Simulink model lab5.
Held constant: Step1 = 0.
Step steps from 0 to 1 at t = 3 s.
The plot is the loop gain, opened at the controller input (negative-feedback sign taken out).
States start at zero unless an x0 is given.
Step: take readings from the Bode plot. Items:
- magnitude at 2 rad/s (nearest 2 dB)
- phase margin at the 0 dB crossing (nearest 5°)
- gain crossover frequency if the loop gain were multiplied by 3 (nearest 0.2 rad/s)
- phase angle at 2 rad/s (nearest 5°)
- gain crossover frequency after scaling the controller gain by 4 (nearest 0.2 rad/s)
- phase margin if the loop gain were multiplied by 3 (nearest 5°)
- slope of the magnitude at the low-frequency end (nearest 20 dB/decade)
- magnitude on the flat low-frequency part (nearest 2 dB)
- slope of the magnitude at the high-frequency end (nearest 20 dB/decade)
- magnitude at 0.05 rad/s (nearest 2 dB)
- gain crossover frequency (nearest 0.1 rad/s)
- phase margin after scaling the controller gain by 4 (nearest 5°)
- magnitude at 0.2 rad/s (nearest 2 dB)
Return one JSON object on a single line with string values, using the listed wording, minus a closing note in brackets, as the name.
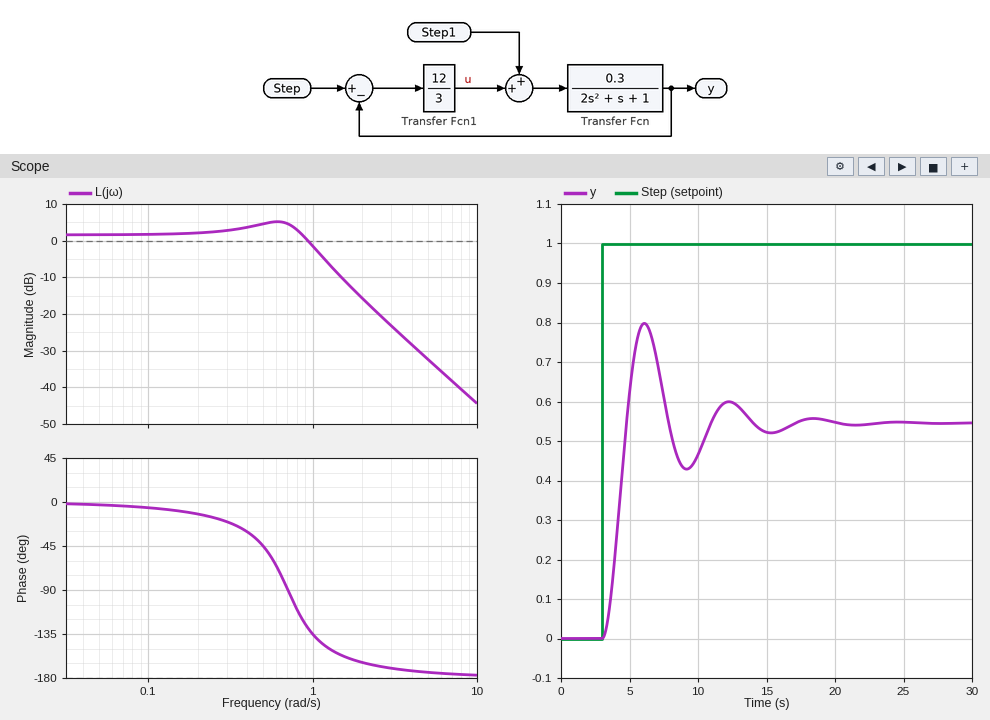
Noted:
{"magnitude at 2 rad/s": "-16 dB", "phase margin at the 0 dB crossing": "50°", "gain crossover frequency if the loop gain were multiplied by 3": "1.4 rad/s", "phase angle at 2 rad/s": "-165°", "gain crossover frequency after scaling the controller gain by 4": "1.6 rad/s", "phase margin if the loop gain were multiplied by 3": "25°", "slope of the magnitude at the low-frequency end": "0 dB/decade", "magnitude on the flat low-frequency part": "2 dB", "slope of the magnitude at the high-frequency end": "-40 dB/decade", "magnitude at 0.05 rad/s": "2 dB", "gain crossover frequency": "0.9 rad/s", "phase margin after scaling the controller gain by 4": "20°", "magnitude at 0.2 rad/s": "2 dB"}
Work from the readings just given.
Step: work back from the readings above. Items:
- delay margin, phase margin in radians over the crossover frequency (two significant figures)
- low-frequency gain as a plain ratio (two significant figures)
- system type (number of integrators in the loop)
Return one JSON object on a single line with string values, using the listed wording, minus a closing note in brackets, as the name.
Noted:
{"delay margin, phase margin in radians over the crossover frequency": "0.97 s", "low-frequency gain as a plain ratio": "1.3", "system type": "0"}
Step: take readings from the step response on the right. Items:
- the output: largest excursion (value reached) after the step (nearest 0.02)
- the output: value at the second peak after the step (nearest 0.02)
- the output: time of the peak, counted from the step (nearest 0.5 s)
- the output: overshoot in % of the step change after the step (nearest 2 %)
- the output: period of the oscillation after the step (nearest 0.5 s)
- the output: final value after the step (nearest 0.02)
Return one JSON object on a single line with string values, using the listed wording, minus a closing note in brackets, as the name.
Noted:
{"the output: largest excursion (value reached) after the step": "0.80", "the output: value at the second peak after the step": "0.60", "the output: time of the peak, counted from the step": "3.0 s", "the output: overshoot in % of the step change after the step": "46 %", "the output: period of the oscillation after the step": "6.0 s", "the output: final value after the step": "0.54"}
